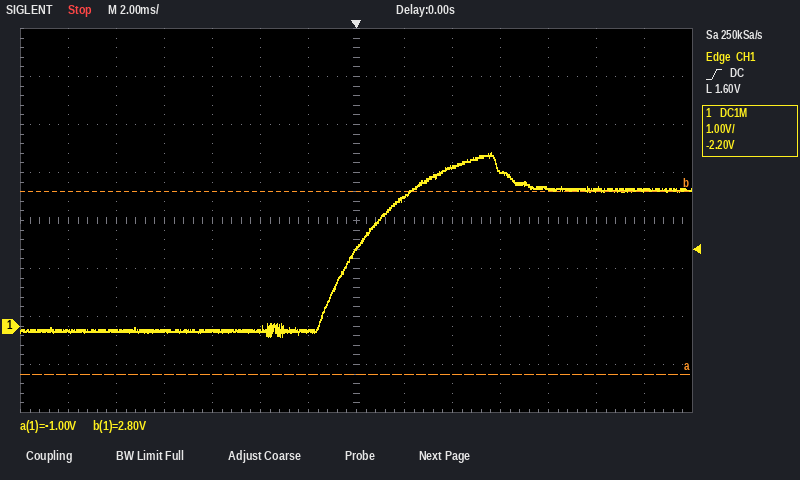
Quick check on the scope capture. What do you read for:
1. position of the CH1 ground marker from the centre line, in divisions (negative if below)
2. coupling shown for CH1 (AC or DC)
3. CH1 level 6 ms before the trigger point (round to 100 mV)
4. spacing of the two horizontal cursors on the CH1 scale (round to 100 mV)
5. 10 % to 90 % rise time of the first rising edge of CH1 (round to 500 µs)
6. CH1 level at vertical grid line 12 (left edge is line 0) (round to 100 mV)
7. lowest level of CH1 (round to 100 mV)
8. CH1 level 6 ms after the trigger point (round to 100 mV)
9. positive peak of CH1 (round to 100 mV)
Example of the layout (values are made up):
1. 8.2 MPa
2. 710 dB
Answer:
1. -2.2 div
2. DC
3. -100 mV
4. 3.8 V
5. 3.0 ms
6. 2.8 V
7. -200 mV
8. 3.2 V
9. 3.6 V
